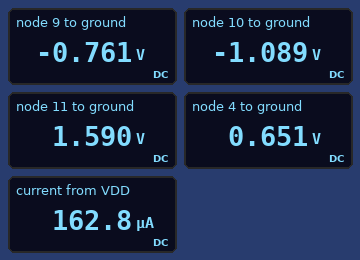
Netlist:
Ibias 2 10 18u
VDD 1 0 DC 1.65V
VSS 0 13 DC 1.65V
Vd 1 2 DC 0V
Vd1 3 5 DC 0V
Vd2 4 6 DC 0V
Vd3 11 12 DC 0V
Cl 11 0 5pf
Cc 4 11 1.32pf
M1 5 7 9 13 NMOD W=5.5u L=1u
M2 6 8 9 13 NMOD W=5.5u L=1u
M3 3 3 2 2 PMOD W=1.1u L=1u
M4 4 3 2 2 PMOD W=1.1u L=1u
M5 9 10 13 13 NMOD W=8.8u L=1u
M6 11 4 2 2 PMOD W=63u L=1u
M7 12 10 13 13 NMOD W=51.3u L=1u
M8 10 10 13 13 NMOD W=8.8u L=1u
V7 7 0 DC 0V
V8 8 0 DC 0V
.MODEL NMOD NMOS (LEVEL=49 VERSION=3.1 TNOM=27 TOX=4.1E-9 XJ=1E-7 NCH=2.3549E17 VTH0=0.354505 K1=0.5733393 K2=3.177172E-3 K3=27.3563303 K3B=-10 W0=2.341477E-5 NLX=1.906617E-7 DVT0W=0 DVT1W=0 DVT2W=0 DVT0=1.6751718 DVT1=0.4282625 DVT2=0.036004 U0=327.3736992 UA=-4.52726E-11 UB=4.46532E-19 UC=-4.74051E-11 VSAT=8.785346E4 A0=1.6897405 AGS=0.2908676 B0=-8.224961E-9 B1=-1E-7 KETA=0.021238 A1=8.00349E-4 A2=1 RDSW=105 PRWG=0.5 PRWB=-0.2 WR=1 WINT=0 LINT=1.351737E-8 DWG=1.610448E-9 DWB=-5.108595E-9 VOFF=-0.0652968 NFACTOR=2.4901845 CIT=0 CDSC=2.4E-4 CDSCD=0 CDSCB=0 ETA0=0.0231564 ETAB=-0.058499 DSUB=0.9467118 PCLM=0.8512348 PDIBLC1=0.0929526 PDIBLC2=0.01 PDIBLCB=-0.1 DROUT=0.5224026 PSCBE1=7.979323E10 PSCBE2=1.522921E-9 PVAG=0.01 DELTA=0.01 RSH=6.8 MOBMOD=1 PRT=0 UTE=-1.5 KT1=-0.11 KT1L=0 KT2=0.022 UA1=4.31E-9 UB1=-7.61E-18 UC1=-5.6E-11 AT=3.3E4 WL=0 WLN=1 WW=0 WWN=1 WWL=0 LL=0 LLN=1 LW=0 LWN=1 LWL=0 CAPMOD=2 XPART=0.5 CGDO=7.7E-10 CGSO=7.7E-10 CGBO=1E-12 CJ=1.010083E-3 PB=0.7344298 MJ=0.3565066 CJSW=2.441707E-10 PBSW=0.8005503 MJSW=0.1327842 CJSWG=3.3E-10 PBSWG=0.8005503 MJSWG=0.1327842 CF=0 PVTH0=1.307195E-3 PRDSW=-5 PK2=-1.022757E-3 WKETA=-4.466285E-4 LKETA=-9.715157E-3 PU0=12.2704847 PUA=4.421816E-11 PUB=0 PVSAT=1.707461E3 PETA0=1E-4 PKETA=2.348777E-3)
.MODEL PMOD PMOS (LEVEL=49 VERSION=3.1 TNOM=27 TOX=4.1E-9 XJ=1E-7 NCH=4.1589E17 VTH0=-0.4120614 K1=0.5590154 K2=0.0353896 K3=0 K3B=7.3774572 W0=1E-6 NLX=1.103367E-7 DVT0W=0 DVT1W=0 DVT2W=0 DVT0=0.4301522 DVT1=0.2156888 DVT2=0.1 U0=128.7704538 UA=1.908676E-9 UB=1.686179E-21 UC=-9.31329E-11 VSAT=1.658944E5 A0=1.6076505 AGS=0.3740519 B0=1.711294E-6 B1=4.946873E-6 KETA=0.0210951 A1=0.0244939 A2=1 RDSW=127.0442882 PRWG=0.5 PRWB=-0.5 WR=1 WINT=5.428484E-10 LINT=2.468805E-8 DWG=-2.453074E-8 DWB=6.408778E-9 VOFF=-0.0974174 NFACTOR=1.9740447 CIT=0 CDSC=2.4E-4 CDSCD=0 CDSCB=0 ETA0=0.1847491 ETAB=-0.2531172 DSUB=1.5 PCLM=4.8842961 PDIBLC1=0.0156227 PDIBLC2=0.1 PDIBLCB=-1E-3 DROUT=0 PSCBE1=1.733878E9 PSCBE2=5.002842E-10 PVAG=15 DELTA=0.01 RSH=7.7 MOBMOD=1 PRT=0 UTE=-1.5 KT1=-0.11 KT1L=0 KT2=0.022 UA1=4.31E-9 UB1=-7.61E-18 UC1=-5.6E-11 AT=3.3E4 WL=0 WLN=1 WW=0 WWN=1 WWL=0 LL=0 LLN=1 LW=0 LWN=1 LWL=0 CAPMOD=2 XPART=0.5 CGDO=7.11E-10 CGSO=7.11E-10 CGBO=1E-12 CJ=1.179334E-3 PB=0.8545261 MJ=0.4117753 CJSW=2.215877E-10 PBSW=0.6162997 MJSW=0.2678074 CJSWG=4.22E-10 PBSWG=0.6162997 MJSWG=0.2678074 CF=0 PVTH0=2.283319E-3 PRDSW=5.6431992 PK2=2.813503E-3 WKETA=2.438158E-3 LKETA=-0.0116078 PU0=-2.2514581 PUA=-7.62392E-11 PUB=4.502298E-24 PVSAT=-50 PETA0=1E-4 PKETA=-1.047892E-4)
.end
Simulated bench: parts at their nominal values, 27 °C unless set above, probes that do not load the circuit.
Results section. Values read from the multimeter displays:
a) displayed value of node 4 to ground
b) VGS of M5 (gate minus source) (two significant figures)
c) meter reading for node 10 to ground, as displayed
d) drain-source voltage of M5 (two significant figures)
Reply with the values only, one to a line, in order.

0.651 V
560 mV
-1.089 V
890 mV
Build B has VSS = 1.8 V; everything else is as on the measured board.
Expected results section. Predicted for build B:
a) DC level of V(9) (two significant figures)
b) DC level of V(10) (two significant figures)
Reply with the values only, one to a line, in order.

-790 mV
-1.2 V
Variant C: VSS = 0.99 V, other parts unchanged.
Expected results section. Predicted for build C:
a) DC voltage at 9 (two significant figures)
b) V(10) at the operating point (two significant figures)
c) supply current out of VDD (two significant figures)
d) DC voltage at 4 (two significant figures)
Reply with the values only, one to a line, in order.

-640 mV
-430 mV
160 µA
660 mV
